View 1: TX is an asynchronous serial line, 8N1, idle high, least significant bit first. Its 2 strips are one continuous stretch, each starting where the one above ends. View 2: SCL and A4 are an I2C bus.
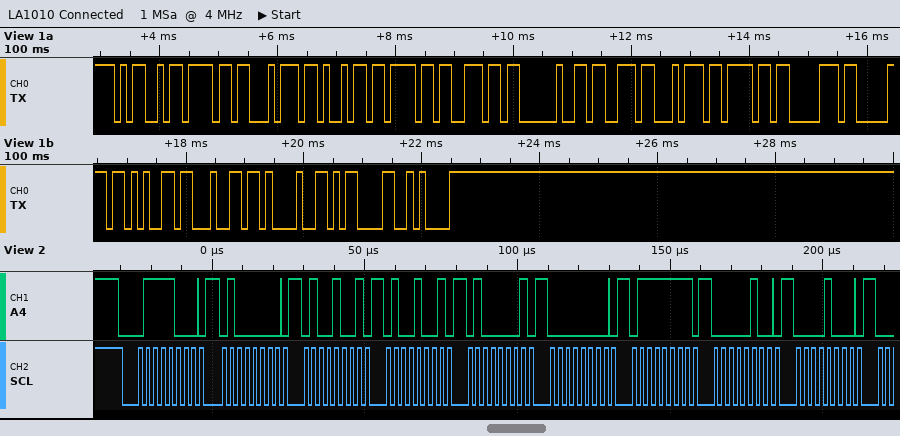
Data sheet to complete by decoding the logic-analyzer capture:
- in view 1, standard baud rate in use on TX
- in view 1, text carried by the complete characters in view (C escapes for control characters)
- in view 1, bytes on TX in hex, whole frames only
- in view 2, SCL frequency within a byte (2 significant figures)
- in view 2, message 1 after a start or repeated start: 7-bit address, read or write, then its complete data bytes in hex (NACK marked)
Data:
9600 baud
"Motion stopped!\r\n"
4D 6F 74 69 6F 6E 20 73 74 6F 70 70 65 64 21 0D 0A
400 kHz
0x3C write: 40 49 49 41 00 7F 04 08
